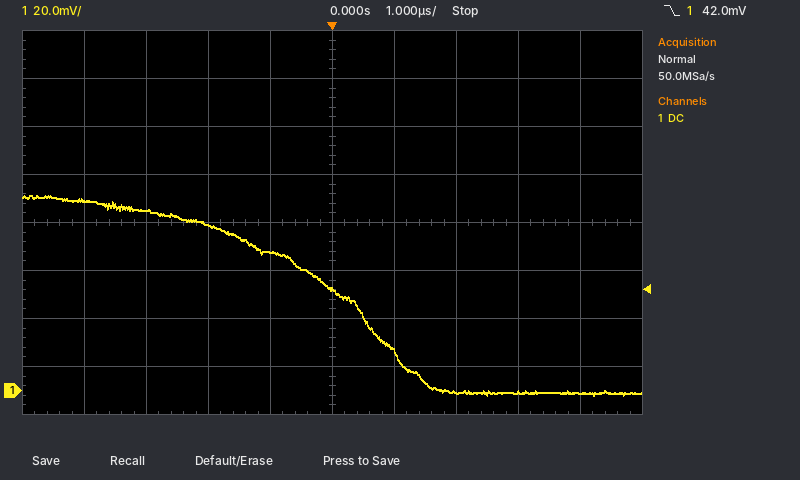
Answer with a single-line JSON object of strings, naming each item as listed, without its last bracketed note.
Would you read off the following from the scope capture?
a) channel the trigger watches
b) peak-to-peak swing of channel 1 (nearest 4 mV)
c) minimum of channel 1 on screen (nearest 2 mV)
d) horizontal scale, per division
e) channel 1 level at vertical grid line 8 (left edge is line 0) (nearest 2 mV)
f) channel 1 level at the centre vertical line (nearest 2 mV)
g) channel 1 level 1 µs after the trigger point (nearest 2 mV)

{"channel the trigger watches": "channel 1", "peak-to-peak swing of channel 1": "84 mV", "minimum of channel 1 on screen": "-2 mV", "horizontal scale, per division": "1 µs", "channel 1 level at vertical grid line 8 (left edge is line 0)": "0 mV", "channel 1 level at the centre vertical line": "42 mV", "channel 1 level 1 µs after the trigger point": "16 mV"}
